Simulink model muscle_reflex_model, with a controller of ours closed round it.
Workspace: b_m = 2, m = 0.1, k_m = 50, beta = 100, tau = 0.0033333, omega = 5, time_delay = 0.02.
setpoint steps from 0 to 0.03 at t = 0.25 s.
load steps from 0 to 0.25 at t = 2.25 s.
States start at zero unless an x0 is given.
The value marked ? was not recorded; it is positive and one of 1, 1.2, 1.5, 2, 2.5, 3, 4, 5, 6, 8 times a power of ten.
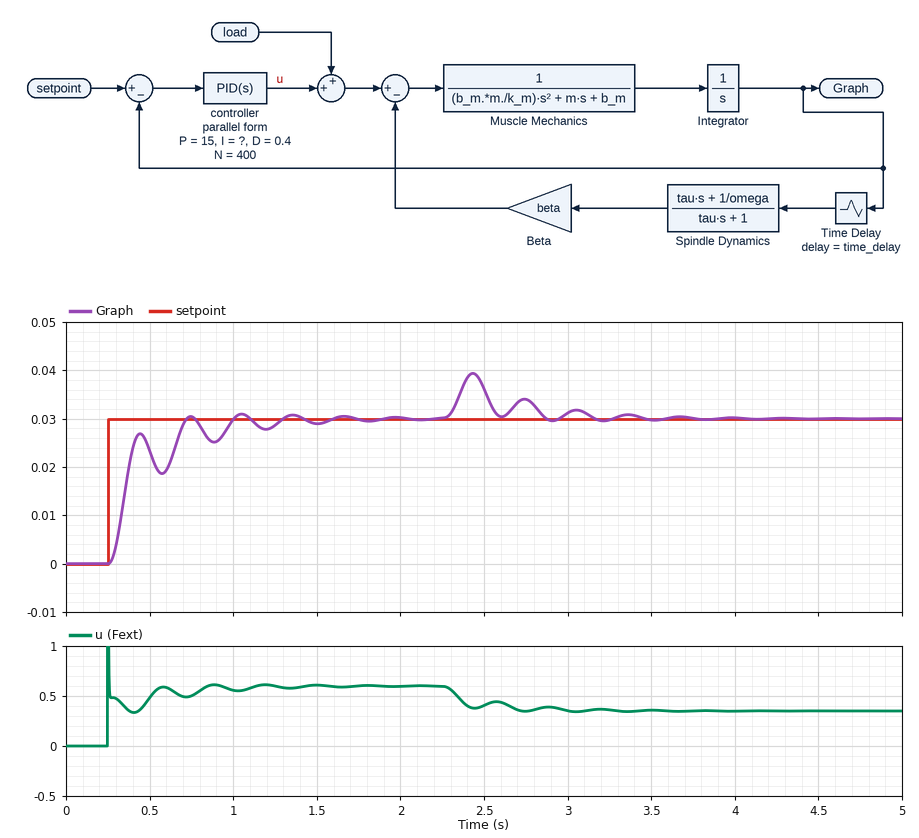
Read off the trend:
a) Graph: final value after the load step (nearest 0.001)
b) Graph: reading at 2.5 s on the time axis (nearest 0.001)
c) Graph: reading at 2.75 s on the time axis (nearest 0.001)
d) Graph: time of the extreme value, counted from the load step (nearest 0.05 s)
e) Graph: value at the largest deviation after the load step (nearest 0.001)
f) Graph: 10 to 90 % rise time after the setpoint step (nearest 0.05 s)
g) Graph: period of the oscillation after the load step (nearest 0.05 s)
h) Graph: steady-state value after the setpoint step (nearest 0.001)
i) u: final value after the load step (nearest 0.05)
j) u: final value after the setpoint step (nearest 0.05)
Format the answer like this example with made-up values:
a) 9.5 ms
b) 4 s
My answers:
a) 0.030
b) 0.036
c) 0.034
d) 0.20 s
e) 0.039
f) 0.40 s
g) 0.30 s
h) 0.030
i) 0.35
j) 0.60
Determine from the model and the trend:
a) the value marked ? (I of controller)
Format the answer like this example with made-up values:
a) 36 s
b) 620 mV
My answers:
a) 100
